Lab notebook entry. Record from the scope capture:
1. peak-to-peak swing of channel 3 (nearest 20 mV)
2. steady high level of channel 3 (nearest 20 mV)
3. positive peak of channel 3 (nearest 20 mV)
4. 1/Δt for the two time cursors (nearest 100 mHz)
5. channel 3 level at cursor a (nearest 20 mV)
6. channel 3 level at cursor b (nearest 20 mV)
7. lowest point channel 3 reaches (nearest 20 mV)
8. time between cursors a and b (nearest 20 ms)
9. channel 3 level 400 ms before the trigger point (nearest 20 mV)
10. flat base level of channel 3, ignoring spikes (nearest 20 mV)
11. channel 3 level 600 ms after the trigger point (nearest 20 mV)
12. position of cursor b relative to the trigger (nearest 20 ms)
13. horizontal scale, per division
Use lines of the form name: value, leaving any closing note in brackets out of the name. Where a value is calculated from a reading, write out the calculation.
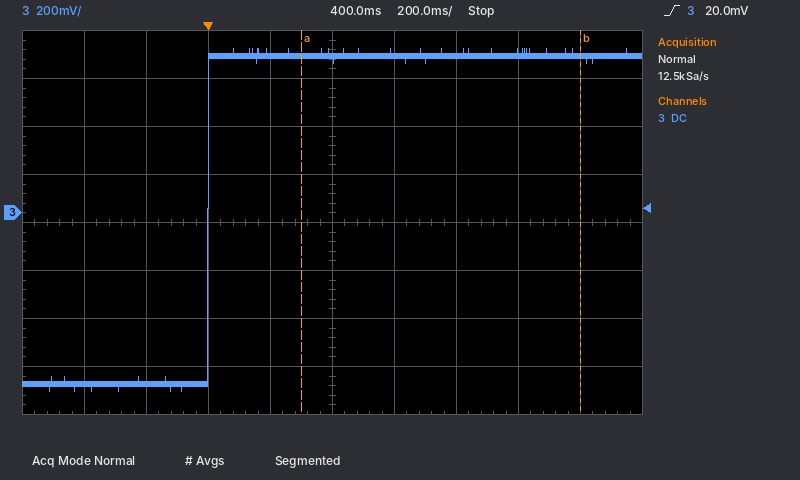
peak-to-peak swing of channel 3: 680 mV − (-740 mV) = 1.42 V
steady high level of channel 3: 660 mV
positive peak of channel 3: 680 mV
1/Δt for the two time cursors: 1 / 900 ms ≈ 1.1 Hz
channel 3 level at cursor a: 660 mV
channel 3 level at cursor b: 660 mV
lowest point channel 3 reaches: -740 mV
time between cursors a and b: 900 ms
channel 3 level 400 ms before the trigger point: -720 mV
flat base level of channel 3, ignoring spikes: -720 mV
channel 3 level 600 ms after the trigger point: 660 mV
position of cursor b relative to the trigger: +1.20 s
horizontal scale, per division: 200 ms
